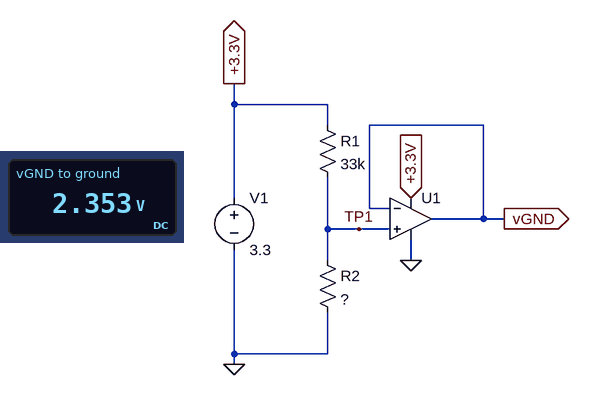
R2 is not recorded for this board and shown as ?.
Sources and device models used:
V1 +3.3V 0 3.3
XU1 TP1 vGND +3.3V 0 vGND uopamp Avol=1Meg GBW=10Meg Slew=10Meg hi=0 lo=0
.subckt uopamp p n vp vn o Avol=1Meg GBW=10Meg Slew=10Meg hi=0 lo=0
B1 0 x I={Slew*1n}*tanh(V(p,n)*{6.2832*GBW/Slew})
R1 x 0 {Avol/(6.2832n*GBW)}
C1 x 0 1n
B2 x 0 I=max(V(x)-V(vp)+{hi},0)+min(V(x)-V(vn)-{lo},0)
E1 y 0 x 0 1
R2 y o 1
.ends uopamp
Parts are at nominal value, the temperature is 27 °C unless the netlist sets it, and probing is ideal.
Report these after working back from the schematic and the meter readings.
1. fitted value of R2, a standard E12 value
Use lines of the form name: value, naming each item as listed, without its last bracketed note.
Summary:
fitted value of R2, a standard E12 value: 82 kΩ
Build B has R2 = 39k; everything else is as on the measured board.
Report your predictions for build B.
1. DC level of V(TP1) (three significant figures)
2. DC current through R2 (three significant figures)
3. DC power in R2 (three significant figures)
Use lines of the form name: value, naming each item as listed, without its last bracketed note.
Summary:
DC level of V(TP1): 1.79 V
DC current through R2: 45.8 µA
DC power in R2: 81.9 µW
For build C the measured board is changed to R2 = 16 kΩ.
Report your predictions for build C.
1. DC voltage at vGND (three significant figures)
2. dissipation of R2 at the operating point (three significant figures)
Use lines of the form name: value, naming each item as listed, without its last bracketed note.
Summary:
DC voltage at vGND: 1.08 V
dissipation of R2 at the operating point: 72.6 µW
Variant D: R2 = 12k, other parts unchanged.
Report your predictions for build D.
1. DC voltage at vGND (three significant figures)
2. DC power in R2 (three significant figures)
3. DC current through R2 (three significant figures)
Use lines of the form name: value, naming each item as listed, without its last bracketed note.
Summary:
DC voltage at vGND: 880 mV
DC power in R2: 64.5 µW
DC current through R2: 73.3 µA
